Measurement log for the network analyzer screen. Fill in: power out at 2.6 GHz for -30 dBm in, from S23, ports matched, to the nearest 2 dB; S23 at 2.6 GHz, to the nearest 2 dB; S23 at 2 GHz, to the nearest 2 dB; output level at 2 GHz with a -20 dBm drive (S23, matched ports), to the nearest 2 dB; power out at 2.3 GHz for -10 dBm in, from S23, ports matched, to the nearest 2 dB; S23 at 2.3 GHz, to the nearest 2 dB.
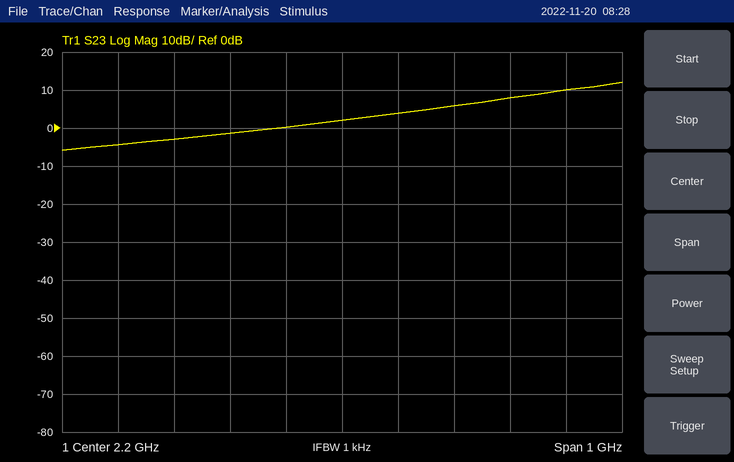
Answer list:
-20 dBm
10 dB
-2 dB
-22 dBm
-6 dBm
4 dB
